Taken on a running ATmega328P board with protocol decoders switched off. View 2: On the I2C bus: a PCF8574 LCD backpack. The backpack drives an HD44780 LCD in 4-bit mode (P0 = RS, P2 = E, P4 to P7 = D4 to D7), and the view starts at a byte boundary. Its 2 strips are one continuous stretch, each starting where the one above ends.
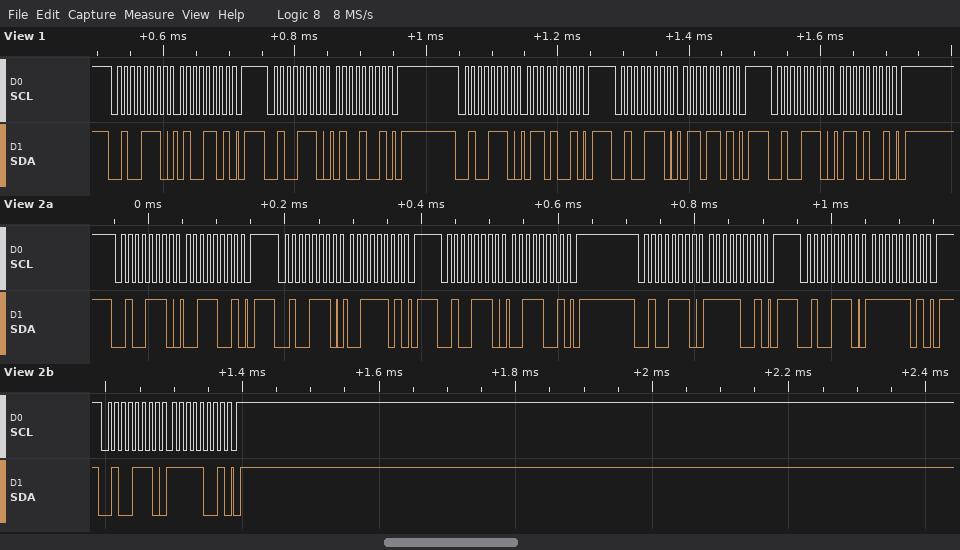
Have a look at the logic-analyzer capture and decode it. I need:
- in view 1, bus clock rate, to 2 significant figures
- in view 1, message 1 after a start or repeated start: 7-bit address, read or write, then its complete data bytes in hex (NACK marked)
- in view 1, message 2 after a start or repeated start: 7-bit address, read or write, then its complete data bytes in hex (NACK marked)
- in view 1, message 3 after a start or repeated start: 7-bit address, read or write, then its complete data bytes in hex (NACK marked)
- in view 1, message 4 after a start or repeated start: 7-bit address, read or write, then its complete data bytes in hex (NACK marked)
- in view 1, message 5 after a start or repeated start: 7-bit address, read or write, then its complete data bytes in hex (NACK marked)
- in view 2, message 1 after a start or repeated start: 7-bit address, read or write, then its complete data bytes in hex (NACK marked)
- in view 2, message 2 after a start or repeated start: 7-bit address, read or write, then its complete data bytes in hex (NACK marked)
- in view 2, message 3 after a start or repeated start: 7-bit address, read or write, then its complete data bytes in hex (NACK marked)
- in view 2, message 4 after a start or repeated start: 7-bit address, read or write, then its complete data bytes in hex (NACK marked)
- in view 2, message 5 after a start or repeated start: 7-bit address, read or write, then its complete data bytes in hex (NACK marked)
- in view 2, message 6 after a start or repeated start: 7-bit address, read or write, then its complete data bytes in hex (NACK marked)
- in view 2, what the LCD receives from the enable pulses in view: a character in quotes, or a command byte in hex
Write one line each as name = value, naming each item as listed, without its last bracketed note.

in view 1, bus clock rate, to 2 significant figures = 100 kHz
in view 1, message 1 after a start or repeated start: 7-bit address, read or write, then its complete data bytes in hex = 0x27 write: 4D
in view 1, message 2 after a start or repeated start: 7-bit address, read or write, then its complete data bytes in hex = 0x27 write: 49
in view 1, message 3 after a start or repeated start: 7-bit address, read or write, then its complete data bytes in hex = 0x27 write: 69
in view 1, message 4 after a start or repeated start: 7-bit address, read or write, then its complete data bytes in hex = 0x27 write: 6D
in view 1, message 5 after a start or repeated start: 7-bit address, read or write, then its complete data bytes in hex = 0x27 write: 69
in view 2, message 1 after a start or repeated start: 7-bit address, read or write, then its complete data bytes in hex = 0x27 write: 39
in view 2, message 2 after a start or repeated start: 7-bit address, read or write, then its complete data bytes in hex = 0x27 write: 3D
in view 2, message 3 after a start or repeated start: 7-bit address, read or write, then its complete data bytes in hex = 0x27 write: 39
in view 2, message 4 after a start or repeated start: 7-bit address, read or write, then its complete data bytes in hex = 0x27 write: F9
in view 2, message 5 after a start or repeated start: 7-bit address, read or write, then its complete data bytes in hex = 0x27 write: FD
in view 2, message 6 after a start or repeated start: 7-bit address, read or write, then its complete data bytes in hex = 0x27 write: F9
in view 2, what the LCD receives from the enable pulses in view: a character in quotes, or a command byte in hex = '?'
